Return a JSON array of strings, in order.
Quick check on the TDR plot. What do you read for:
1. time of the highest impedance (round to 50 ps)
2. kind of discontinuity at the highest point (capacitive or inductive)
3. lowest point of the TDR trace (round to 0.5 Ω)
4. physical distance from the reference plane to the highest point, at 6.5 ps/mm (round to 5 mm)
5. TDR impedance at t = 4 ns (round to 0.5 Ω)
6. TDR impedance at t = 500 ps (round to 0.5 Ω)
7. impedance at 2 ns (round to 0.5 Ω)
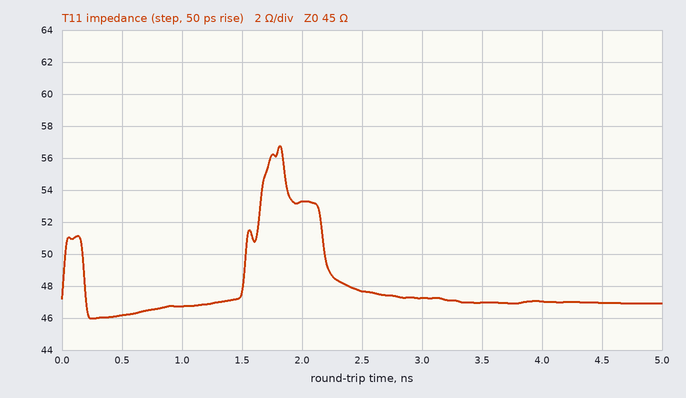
["1.80 ns", "inductive", "46.0 Ω", "140 mm", "47.0 Ω", "46.0 Ω", "53.5 Ω"]
